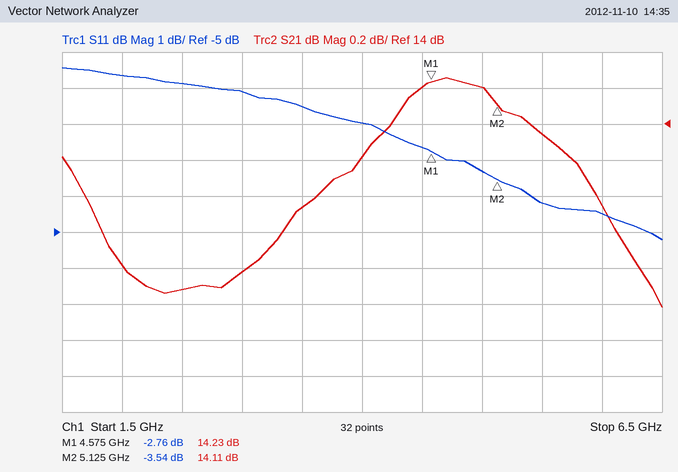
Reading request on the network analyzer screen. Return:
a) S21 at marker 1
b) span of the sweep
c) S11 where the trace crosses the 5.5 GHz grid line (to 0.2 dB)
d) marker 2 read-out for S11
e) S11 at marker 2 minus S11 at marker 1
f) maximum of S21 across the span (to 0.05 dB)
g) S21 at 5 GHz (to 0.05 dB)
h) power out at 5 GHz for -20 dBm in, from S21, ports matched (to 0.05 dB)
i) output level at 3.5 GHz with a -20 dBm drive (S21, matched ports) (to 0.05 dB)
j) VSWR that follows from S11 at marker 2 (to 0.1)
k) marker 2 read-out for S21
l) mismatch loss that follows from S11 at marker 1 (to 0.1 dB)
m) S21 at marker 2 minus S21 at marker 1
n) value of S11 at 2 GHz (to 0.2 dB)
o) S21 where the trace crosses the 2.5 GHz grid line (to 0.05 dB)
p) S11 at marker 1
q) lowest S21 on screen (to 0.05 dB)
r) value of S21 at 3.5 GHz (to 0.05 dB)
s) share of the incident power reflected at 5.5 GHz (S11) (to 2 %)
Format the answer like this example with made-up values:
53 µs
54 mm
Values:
14.23 dB
5 GHz
-4.2 dB
-3.54 dB
-0.78 dB
14.25 dB
14.20 dB
-5.80 dBm
-6.45 dBm
5.0
14.11 dB
3.3 dB
-0.12 dB
-0.6 dB
13.10 dB
-2.76 dB
13.00 dB
13.55 dB
38 %
